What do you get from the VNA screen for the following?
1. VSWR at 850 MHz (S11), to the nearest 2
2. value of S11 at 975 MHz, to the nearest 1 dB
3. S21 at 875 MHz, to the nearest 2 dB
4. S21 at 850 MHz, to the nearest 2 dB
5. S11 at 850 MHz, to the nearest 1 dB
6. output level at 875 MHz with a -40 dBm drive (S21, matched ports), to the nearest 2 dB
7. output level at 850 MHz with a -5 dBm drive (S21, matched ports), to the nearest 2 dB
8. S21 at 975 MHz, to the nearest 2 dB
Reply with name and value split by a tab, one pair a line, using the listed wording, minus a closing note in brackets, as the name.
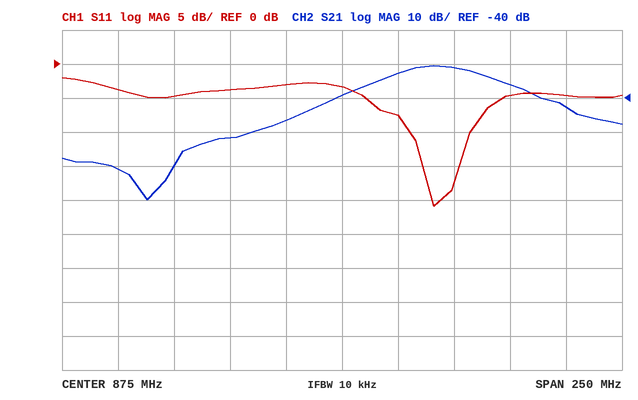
VSWR at 850 MHz (S11), to the nearest 2	6
value of S11 at 975 MHz, to the nearest 1 dB	-5 dB
S21 at 875 MHz, to the nearest 2 dB	-40 dB
S21 at 850 MHz, to the nearest 2 dB	-46 dB
S11 at 850 MHz, to the nearest 1 dB	-3 dB
output level at 875 MHz with a -40 dBm drive (S21, matched ports), to the nearest 2 dB	-80 dBm
output level at 850 MHz with a -5 dBm drive (S21, matched ports), to the nearest 2 dB	-52 dBm
S21 at 975 MHz, to the nearest 2 dB	-42 dB
